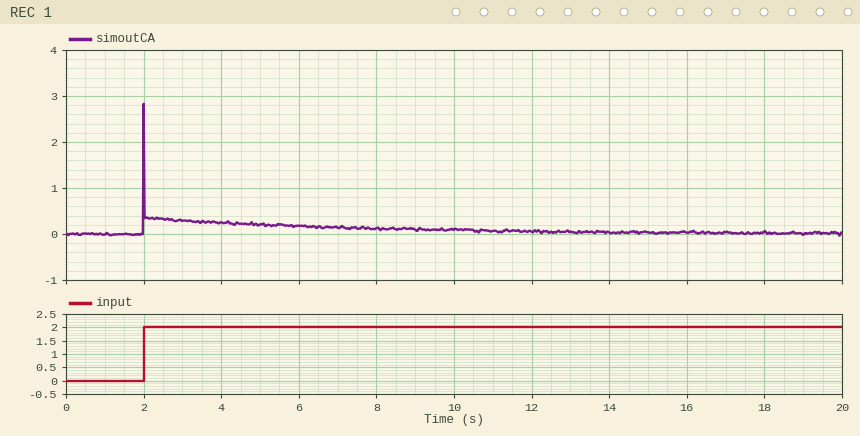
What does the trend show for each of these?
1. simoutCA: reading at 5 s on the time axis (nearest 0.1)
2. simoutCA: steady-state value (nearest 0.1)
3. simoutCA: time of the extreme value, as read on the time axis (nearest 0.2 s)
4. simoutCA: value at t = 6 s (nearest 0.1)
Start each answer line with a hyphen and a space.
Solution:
- 0.2
- 0.0
- 2.0 s
- 0.2
